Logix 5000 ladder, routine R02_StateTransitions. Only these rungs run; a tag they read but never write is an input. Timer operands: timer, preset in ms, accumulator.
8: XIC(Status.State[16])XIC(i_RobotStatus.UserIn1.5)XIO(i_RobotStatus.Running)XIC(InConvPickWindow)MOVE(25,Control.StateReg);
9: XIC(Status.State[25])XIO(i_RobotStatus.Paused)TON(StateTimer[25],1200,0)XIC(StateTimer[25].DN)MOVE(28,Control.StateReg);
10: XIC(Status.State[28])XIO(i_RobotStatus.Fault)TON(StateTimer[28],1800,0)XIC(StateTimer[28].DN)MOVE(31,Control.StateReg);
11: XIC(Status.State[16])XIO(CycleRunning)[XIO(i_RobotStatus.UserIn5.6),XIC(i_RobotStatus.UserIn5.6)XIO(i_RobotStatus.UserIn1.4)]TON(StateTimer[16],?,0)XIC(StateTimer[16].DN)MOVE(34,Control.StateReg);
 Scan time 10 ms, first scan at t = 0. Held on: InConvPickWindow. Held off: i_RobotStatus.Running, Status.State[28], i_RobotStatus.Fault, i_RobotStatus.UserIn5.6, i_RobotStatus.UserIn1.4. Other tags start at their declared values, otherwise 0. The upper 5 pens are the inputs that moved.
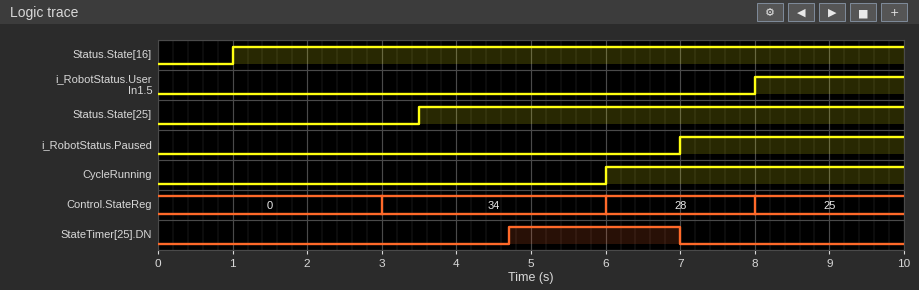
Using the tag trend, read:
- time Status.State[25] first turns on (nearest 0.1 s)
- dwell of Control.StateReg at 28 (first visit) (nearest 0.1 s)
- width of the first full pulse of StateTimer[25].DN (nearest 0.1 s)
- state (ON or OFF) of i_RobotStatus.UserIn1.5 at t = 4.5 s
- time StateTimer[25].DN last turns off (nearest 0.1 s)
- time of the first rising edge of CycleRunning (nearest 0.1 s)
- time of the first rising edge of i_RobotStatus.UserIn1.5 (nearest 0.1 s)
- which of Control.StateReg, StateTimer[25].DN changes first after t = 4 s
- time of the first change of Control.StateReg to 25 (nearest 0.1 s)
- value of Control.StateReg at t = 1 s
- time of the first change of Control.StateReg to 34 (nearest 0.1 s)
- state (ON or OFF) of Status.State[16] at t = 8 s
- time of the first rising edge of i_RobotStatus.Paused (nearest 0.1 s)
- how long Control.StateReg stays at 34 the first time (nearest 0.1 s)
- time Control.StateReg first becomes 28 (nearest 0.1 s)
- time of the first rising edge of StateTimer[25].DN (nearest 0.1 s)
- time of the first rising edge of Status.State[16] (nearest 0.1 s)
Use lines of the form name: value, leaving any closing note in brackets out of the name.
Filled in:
time Status.State[25] first turns on: 3.5 s
dwell of Control.StateReg at 28 (first visit): 2.0 s
width of the first full pulse of StateTimer[25].DN: 2.3 s
state (ON or OFF) of i_RobotStatus.UserIn1.5 at t = 4.5 s: OFF
time StateTimer[25].DN last turns off: 7.0 s
time of the first rising edge of CycleRunning: 6.0 s
time of the first rising edge of i_RobotStatus.UserIn1.5: 8.0 s
which of Control.StateReg, StateTimer[25].DN changes first after t = 4 s: StateTimer[25].DN
time of the first change of Control.StateReg to 25: 8.0 s
value of Control.StateReg at t = 1 s: 0
time of the first change of Control.StateReg to 34: 3.0 s
state (ON or OFF) of Status.State[16] at t = 8 s: ON
time of the first rising edge of i_RobotStatus.Paused: 7.0 s
how long Control.StateReg stays at 34 the first time: 3.0 s
time Control.StateReg first becomes 28: 6.0 s
time of the first rising edge of StateTimer[25].DN: 4.7 s
time of the first rising edge of Status.State[16]: 1.0 s
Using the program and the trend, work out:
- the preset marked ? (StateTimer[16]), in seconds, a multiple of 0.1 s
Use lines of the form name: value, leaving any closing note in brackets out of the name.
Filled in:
the preset marked ? (StateTimer[16]), in seconds, a multiple of 0.1 s: 2.0 s
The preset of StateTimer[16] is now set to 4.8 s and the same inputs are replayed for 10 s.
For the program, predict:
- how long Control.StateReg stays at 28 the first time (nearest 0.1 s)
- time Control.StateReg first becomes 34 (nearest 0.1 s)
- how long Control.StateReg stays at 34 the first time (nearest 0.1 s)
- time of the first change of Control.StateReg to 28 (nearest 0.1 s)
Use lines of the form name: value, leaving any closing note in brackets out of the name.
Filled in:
how long Control.StateReg stays at 28 the first time: 1.1 s
time Control.StateReg first becomes 34: 5.8 s
how long Control.StateReg stays at 34 the first time: 0.2 s
time of the first change of Control.StateReg to 28: 4.7 s
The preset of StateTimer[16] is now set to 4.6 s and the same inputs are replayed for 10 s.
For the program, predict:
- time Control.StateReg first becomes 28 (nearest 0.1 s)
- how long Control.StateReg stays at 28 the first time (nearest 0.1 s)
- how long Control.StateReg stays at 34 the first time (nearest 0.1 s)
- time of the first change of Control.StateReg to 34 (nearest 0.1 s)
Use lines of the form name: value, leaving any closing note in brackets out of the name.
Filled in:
time Control.StateReg first becomes 28: 4.7 s
how long Control.StateReg stays at 28 the first time: 0.9 s
how long Control.StateReg stays at 34 the first time: 0.4 s
time of the first change of Control.StateReg to 34: 5.6 s
